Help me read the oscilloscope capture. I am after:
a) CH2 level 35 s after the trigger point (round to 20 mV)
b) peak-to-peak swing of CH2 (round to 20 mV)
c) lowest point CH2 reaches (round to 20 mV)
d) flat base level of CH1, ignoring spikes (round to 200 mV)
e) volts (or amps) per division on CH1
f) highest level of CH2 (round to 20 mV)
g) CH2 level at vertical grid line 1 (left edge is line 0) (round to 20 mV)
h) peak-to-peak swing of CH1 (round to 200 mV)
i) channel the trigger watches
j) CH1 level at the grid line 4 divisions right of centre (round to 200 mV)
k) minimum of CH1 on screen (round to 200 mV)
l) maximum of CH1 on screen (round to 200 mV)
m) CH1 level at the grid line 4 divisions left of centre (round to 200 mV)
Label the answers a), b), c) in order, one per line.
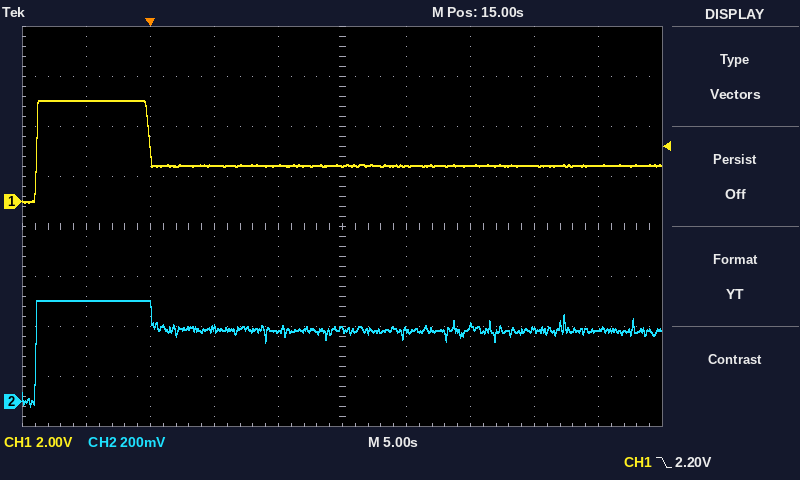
a) 280 mV
b) 420 mV
c) -20 mV
d) 1.4 V
e) 2 V
f) 400 mV
g) 400 mV
h) 4.0 V
i) CH1
j) 1.4 V
k) 0.0 V
l) 4.0 V
m) 4.0 V
